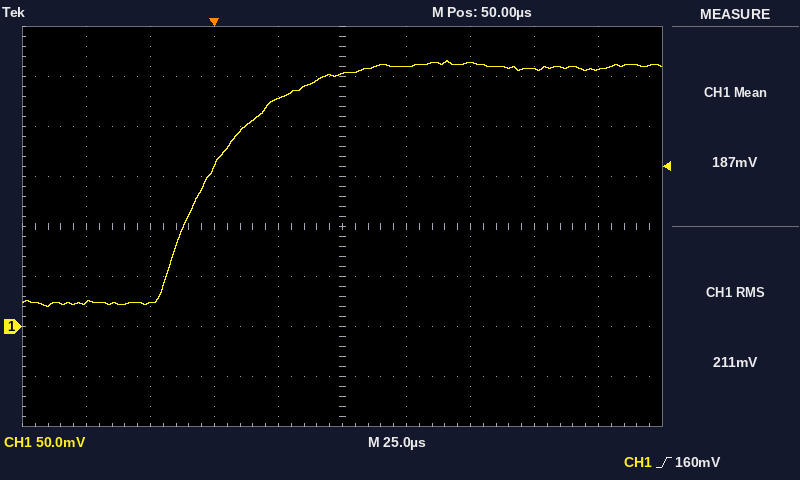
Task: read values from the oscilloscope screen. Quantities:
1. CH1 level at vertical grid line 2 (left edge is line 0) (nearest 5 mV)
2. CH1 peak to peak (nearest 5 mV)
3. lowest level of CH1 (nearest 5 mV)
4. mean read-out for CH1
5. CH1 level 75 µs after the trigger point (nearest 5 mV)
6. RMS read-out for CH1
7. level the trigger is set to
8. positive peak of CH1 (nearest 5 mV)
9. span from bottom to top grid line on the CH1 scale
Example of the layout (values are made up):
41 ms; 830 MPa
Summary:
25 mV; 245 mV; 20 mV; 187 mV; 260 mV; 211 mV; 160 mV; 265 mV; 400 mV
